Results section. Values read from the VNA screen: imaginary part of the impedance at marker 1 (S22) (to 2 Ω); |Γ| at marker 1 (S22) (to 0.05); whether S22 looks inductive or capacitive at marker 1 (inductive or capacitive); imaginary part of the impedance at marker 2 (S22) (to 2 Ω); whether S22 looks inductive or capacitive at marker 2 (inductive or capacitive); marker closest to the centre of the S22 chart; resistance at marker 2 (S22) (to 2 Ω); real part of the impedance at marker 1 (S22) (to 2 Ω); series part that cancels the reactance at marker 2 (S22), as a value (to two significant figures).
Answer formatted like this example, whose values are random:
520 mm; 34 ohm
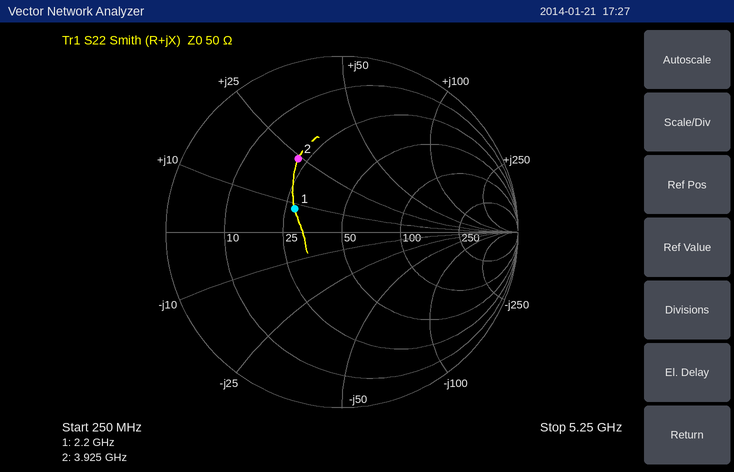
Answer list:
+8 Ω; 0.30; inductive; +24 Ω; inductive; marker 1; 22 Ω; 28 Ω; 1.7 pF
